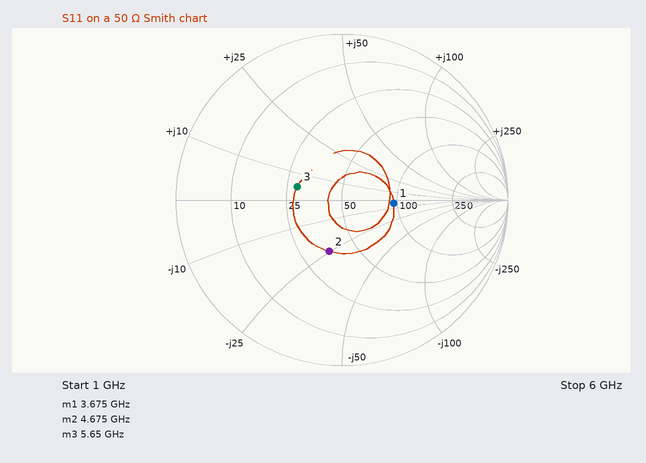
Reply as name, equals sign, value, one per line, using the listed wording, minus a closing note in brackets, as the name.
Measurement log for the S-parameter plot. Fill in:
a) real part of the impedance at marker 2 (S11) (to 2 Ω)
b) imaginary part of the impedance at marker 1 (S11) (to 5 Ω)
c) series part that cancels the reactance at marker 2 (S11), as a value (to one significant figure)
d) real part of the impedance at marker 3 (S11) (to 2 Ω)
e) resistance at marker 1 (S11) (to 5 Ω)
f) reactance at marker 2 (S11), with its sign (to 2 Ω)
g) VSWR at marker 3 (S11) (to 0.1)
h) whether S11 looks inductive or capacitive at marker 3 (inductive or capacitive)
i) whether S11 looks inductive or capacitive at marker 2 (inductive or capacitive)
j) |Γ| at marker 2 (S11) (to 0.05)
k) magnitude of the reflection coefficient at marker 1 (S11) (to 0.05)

real part of the impedance at marker 2 (S11) = 36 Ω
imaginary part of the impedance at marker 1 (S11) = -5 Ω
series part that cancels the reactance at marker 2 (S11), as a value = 800 pH
real part of the impedance at marker 3 (S11) = 28 Ω
resistance at marker 1 (S11) = 95 Ω
reactance at marker 2 (S11), with its sign = -24 Ω
VSWR at marker 3 (S11) = 1.8
whether S11 looks inductive or capacitive at marker 3 = inductive
whether S11 looks inductive or capacitive at marker 2 = capacitive
|Γ| at marker 2 (S11) = 0.30
magnitude of the reflection coefficient at marker 1 (S11) = 0.30
